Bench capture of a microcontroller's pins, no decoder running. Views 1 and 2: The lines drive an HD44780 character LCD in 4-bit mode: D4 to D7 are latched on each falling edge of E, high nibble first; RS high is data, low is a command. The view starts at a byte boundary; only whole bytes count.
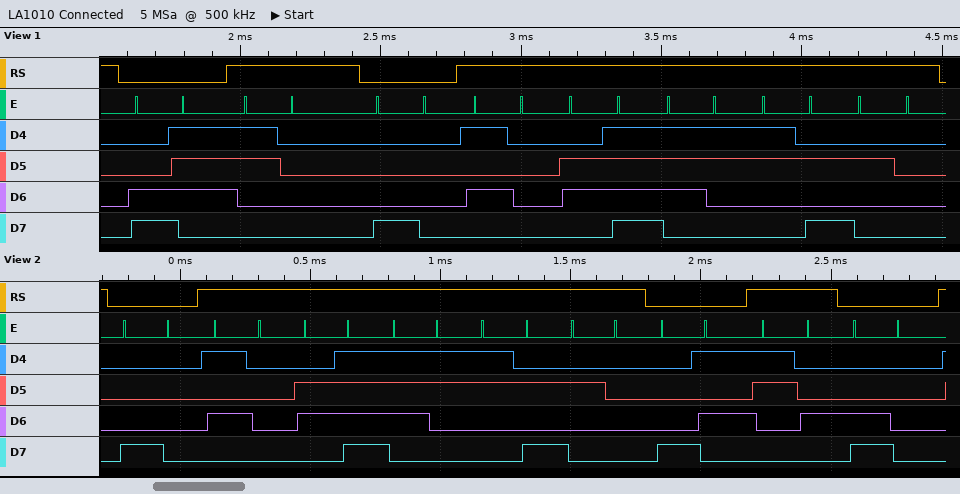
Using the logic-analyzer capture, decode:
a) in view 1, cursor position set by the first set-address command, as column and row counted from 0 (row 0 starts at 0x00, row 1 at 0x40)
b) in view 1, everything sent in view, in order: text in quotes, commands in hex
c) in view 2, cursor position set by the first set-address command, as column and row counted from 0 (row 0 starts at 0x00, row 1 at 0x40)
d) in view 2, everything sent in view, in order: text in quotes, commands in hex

column 7, row 1
0xC7 "0" 0x80 "Pos: "
column 0, row 0
0x80 "Pos: " 0x85 "4" 0xC0
